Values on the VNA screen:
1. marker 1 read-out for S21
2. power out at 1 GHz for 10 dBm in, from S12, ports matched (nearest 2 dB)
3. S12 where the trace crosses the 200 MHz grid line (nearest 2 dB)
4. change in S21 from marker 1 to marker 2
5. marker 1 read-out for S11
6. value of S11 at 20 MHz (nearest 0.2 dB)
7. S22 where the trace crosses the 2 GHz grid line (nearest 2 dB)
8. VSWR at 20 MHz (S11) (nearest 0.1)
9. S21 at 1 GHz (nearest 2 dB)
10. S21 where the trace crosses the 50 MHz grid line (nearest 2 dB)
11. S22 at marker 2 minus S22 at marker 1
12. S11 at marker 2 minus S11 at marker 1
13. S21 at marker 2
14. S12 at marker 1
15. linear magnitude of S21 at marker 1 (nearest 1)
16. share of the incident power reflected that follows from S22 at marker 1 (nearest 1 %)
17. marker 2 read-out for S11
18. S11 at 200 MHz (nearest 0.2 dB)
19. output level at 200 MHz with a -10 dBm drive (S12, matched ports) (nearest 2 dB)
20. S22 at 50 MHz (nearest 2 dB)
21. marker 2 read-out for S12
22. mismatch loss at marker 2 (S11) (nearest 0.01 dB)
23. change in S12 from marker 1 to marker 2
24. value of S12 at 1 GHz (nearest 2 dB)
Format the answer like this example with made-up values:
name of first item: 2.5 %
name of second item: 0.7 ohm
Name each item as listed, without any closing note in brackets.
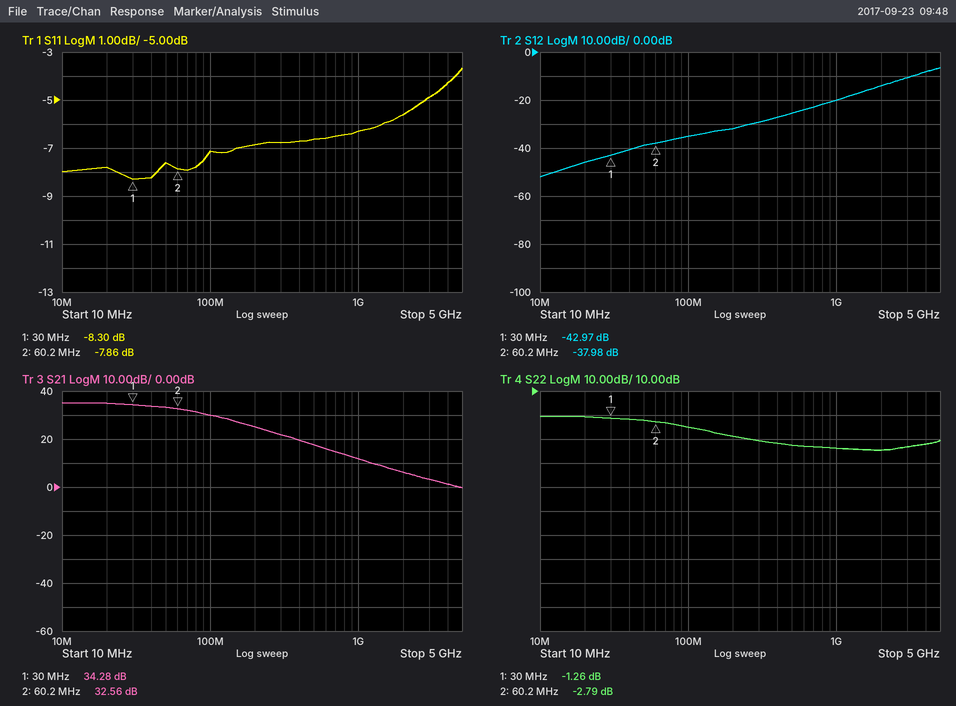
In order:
marker 1 read-out for S21: 34.28 dB
power out at 1 GHz for 10 dBm in, from S12, ports matched: -10 dBm
S12 where the trace crosses the 200 MHz grid line: -32 dB
change in S21 from marker 1 to marker 2: -1.72 dB
marker 1 read-out for S11: -8.30 dB
value of S11 at 20 MHz: -7.8 dB
S22 where the trace crosses the 2 GHz grid line: -14 dB
VSWR at 20 MHz (S11): 2.4
S21 at 1 GHz: 12 dB
S21 where the trace crosses the 50 MHz grid line: 34 dB
S22 at marker 2 minus S22 at marker 1: -1.53 dB
S11 at marker 2 minus S11 at marker 1: 0.44 dB
S21 at marker 2: 32.56 dB
S12 at marker 1: -42.97 dB
linear magnitude of S21 at marker 1: 52
share of the incident power reflected that follows from S22 at marker 1: 75 %
marker 2 read-out for S11: -7.86 dB
S11 at 200 MHz: -6.8 dB
output level at 200 MHz with a -10 dBm drive (S12, matched ports): -42 dBm
S22 at 50 MHz: -2 dB
marker 2 read-out for S12: -37.98 dB
mismatch loss at marker 2 (S11): 0.78 dB
change in S12 from marker 1 to marker 2: 4.99 dB
value of S12 at 1 GHz: -20 dB
